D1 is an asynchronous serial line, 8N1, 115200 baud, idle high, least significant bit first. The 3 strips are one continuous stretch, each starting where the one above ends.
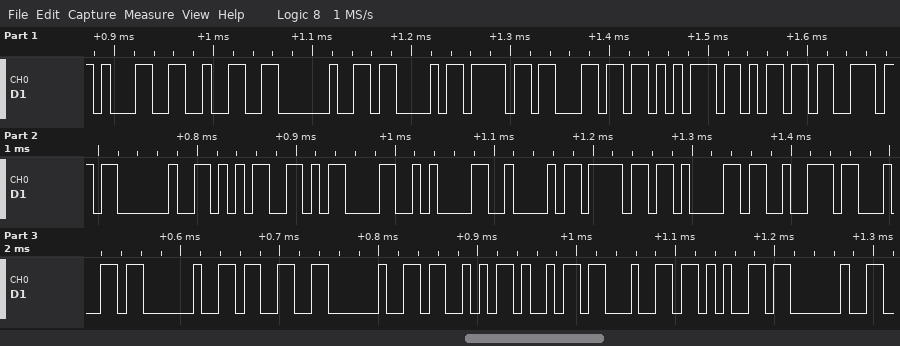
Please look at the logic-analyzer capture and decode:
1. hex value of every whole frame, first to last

31 32 20 43 6F 6C 75 6D 6E 20 35 0D 0A 42 6F 61 72 64 20 33 20 53 69 64 65 20
